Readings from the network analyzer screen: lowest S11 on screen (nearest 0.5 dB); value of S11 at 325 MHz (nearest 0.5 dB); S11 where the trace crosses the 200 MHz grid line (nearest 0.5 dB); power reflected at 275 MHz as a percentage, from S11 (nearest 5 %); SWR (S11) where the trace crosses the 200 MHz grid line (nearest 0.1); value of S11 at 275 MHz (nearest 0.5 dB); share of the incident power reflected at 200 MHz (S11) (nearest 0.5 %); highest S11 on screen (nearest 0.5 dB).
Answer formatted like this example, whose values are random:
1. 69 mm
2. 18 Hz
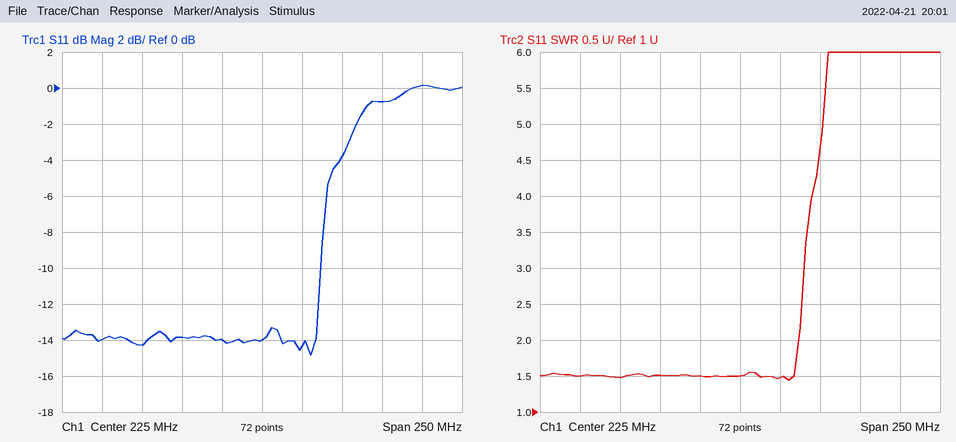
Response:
1. -15.0 dB
2. 0.0 dB
3. -14.0 dB
4. 40 %
5. 1.5
6. -4.0 dB
7. 4.0 %
8. 0.0 dB
